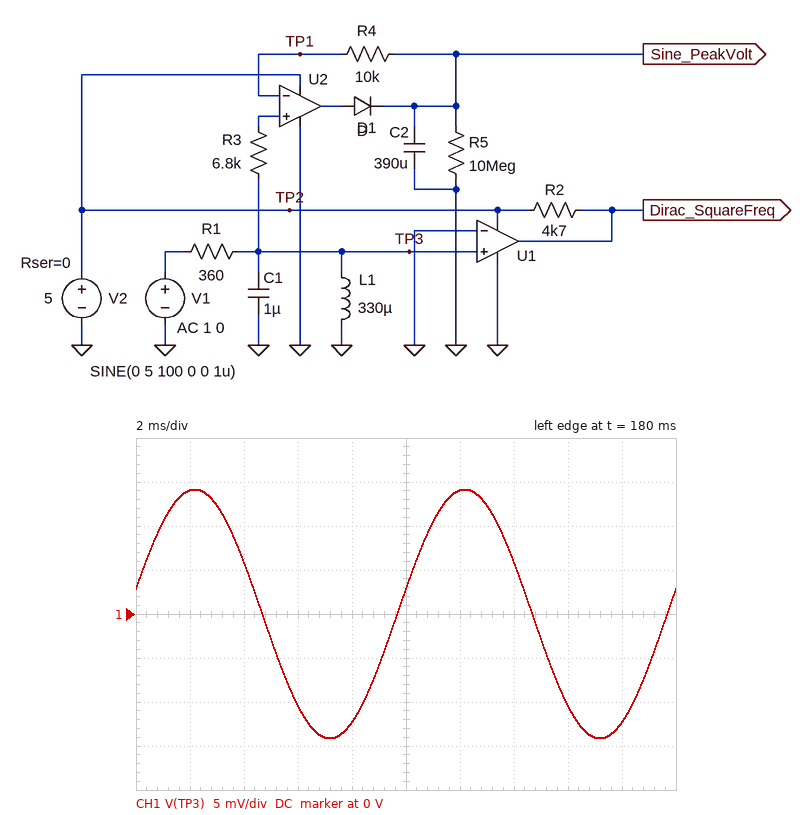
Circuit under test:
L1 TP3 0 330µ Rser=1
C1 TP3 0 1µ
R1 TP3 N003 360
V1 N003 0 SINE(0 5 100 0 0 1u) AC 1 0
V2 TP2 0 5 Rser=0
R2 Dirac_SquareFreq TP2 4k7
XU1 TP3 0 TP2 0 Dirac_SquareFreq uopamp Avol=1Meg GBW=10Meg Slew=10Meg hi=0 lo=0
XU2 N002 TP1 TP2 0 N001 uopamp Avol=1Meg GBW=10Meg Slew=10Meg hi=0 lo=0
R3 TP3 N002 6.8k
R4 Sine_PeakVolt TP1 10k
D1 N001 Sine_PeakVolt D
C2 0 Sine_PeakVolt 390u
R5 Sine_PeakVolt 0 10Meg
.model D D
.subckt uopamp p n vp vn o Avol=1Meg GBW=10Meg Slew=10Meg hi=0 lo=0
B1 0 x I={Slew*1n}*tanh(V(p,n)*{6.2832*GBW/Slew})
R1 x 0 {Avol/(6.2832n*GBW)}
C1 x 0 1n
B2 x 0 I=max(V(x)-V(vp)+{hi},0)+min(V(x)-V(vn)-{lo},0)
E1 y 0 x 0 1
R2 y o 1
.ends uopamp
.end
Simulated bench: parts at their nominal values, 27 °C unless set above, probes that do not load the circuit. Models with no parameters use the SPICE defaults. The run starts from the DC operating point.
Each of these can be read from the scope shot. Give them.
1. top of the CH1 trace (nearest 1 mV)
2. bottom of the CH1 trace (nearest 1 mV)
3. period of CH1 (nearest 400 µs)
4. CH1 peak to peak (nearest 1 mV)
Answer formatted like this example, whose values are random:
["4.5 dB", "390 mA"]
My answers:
["14 mV", "-14 mV", "10.0 ms", "28 mV"]
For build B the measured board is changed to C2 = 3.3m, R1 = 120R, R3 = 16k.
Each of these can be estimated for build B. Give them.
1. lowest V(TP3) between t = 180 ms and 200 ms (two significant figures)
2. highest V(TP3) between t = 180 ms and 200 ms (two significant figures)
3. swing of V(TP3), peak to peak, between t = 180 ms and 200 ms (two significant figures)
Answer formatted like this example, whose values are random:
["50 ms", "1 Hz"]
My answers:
["-42 mV", "42 mV", "84 mV"]
